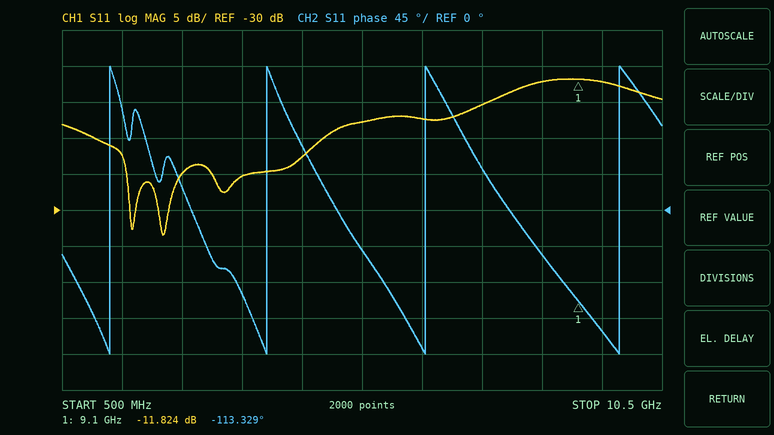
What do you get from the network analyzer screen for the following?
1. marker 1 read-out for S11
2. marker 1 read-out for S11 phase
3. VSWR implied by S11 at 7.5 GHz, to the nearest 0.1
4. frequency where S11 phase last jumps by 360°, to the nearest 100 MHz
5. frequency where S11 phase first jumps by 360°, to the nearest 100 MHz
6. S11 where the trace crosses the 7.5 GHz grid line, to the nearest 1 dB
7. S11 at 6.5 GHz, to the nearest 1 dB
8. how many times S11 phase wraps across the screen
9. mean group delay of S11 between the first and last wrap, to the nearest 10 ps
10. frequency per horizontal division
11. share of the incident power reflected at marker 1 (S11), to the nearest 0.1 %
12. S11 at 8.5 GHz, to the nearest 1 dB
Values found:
-11.824 dB
-113.329°
1.4
9.8 GHz
1.3 GHz
-15 dB
-17 dB
4
350 ps
1 GHz
6.6 %
-12 dB
